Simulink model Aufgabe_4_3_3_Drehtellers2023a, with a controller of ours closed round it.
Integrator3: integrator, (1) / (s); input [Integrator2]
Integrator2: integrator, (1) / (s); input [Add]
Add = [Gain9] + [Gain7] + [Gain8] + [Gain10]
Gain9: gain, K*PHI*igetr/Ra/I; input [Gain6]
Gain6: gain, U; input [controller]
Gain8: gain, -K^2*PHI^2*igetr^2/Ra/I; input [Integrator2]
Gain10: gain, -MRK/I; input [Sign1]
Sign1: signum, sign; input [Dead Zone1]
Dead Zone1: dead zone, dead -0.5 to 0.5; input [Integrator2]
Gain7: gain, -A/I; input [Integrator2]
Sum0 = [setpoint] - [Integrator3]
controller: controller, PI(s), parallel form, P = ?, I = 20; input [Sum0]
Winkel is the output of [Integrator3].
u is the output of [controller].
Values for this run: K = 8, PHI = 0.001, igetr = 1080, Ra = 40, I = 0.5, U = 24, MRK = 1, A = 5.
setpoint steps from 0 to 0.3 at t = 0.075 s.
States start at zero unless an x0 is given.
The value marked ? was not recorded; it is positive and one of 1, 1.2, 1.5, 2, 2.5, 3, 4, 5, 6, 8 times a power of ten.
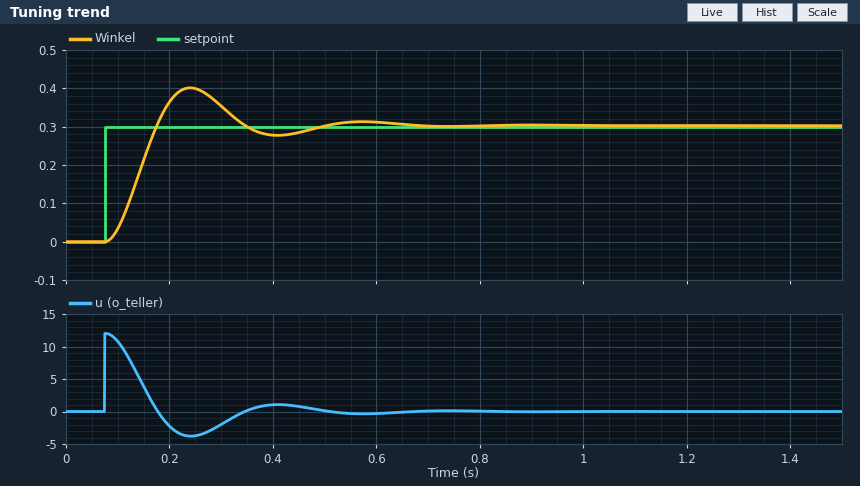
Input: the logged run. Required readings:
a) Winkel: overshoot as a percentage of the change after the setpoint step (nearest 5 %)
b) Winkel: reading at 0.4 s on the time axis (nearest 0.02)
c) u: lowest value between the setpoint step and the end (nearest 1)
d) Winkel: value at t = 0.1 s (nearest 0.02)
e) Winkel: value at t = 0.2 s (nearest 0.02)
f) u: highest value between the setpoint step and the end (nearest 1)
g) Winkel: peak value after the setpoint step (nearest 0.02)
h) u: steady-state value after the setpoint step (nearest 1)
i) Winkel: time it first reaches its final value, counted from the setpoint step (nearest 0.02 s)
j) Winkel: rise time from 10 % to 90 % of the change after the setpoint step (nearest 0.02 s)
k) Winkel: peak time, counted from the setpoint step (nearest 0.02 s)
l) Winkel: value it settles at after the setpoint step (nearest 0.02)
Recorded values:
35 %
0.28
-4
0.04
0.36
12
0.40
0
0.10 s
0.06 s
0.16 s
0.30
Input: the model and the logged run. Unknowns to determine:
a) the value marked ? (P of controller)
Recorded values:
40
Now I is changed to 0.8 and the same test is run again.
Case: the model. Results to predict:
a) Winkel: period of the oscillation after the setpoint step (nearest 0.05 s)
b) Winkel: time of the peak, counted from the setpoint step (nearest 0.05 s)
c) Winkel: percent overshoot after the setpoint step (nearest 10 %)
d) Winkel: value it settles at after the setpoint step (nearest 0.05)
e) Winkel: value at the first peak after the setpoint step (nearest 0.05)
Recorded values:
0.40 s
0.20 s
40 %
0.30
0.45
